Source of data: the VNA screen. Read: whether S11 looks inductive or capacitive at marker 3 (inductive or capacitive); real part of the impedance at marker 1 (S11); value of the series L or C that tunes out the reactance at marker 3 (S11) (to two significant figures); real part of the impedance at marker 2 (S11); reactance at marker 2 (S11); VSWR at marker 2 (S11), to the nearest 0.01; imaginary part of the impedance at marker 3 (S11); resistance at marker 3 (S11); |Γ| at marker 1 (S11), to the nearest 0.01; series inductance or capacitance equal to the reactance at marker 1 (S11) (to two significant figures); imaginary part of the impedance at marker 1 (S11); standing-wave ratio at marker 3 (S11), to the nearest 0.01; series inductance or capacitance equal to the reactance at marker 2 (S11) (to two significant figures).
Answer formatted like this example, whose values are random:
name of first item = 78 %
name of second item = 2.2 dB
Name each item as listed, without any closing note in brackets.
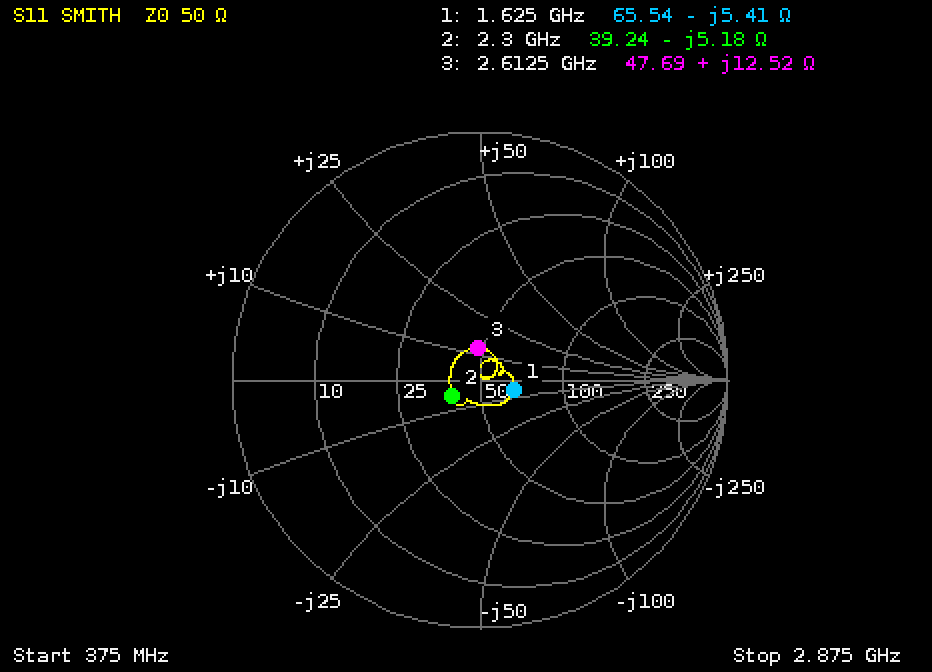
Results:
whether S11 looks inductive or capacitive at marker 3 = inductive
real part of the impedance at marker 1 = 65.54 Ω
value of the series L or C that tunes out the reactance at marker 3 (S11) = 4.9 pF
real part of the impedance at marker 2 = 39.24 Ω
reactance at marker 2 = -5.18 Ω
VSWR at marker 2 (S11), to the nearest 0.01 = 1.31
imaginary part of the impedance at marker 3 = +12.52 Ω
resistance at marker 3 = 47.69 Ω
|Γ| at marker 1 (S11), to the nearest 0.01 = 0.14
series inductance or capacitance equal to the reactance at marker 1 (S11) = 18 pF
imaginary part of the impedance at marker 1 = -5.41 Ω
standing-wave ratio at marker 3 (S11), to the nearest 0.01 = 1.30
series inductance or capacitance equal to the reactance at marker 2 (S11) = 13 pF
